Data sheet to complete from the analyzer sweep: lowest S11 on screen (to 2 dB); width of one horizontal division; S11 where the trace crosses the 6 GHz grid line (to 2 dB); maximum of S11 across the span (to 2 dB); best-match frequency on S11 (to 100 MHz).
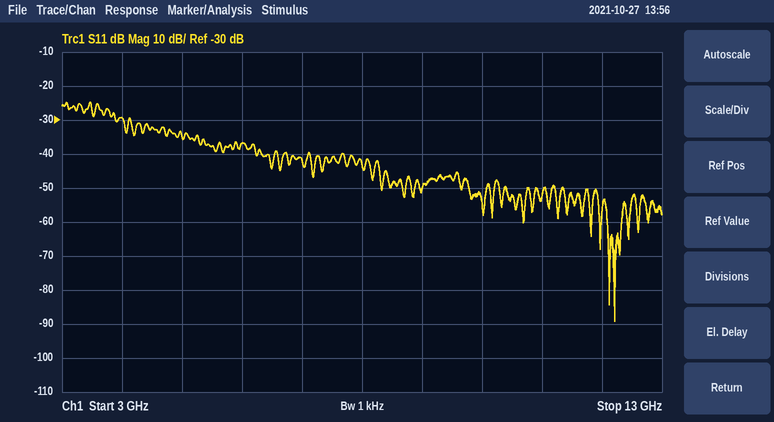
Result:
-90 dB
1 GHz
-36 dB
-24 dB
12.2 GHz
